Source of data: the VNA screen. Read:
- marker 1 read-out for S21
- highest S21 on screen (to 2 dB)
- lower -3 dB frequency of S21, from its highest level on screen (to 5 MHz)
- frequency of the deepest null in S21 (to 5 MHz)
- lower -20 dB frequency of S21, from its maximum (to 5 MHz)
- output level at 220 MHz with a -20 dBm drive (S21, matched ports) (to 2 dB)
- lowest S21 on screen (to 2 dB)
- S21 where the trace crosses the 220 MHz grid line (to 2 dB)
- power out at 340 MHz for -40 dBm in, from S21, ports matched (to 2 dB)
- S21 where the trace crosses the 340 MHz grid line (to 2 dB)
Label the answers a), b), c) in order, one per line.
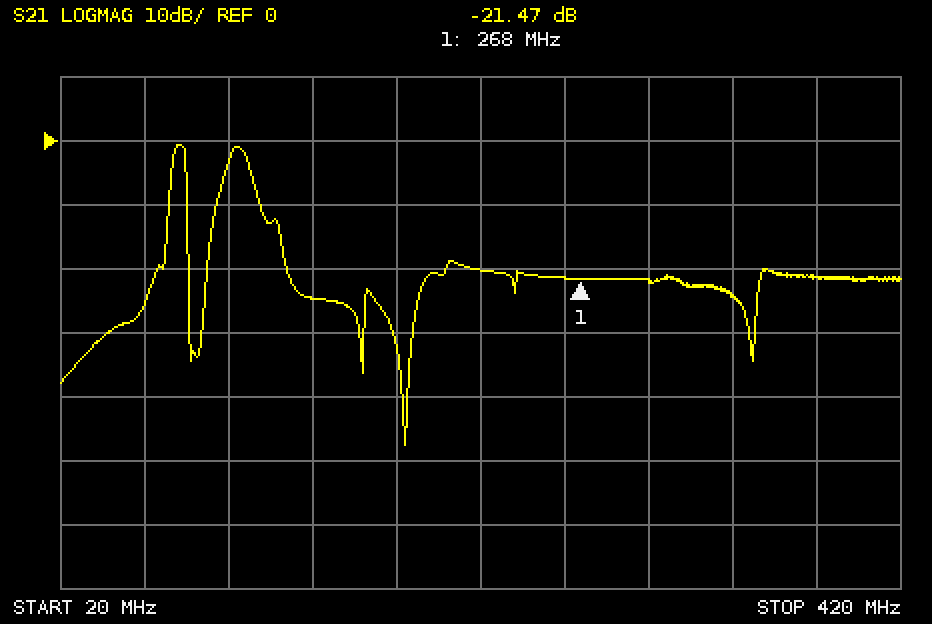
a) -21.47 dB
b) 0 dB
c) 75 MHz
d) 185 MHz
e) 65 MHz
f) -40 dBm
g) -48 dB
h) -20 dB
i) -64 dBm
j) -24 dB
